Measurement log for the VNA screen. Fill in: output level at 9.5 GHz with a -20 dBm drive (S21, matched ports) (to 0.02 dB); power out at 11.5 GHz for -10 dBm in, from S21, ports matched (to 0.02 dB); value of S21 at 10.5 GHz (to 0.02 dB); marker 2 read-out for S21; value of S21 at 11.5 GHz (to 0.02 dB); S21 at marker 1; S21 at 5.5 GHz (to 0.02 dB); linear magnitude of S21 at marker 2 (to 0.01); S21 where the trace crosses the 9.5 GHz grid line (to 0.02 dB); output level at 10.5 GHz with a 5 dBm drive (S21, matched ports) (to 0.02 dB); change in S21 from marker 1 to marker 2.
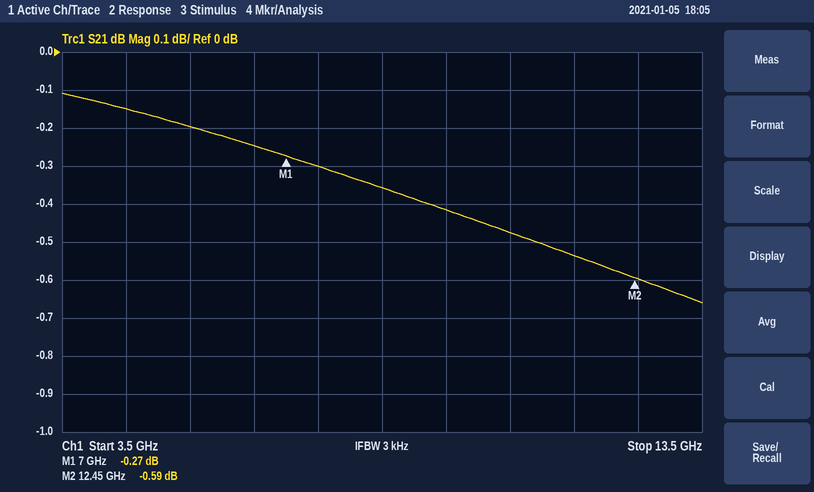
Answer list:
-20.42 dBm
-10.54 dBm
-0.48 dB
-0.59 dB
-0.54 dB
-0.27 dB
-0.20 dB
0.93
-0.42 dB
4.52 dBm
-0.32 dB
